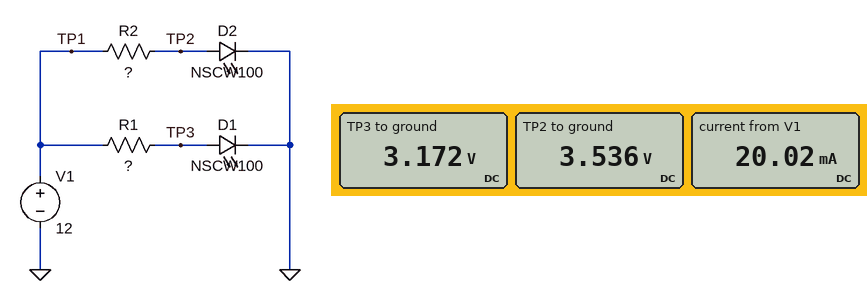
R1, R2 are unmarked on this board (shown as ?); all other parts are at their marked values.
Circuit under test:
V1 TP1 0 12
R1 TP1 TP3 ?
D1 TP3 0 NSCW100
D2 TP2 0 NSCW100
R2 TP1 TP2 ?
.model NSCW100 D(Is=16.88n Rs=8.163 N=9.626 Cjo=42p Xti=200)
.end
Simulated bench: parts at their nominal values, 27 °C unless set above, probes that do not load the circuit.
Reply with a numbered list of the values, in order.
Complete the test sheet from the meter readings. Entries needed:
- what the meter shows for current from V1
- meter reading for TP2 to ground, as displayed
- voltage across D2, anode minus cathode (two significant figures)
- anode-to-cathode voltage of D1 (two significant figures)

1. 20.02 mA
2. 3.536 V
3. 3.5 V
4. 3.2 V
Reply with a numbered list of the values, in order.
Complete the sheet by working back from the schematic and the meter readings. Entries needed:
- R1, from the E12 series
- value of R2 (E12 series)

1. 1.8 kΩ
2. 560 Ω
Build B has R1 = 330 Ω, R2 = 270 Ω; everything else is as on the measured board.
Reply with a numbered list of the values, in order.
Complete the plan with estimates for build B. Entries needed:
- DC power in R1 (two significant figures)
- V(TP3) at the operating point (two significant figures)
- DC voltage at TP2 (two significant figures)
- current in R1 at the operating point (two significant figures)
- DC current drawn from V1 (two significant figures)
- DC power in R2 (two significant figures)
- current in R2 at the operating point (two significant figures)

1. 210 mW
2. 3.7 V
3. 3.8 V
4. 25 mA
5. 55 mA
6. 250 mW
7. 30 mA
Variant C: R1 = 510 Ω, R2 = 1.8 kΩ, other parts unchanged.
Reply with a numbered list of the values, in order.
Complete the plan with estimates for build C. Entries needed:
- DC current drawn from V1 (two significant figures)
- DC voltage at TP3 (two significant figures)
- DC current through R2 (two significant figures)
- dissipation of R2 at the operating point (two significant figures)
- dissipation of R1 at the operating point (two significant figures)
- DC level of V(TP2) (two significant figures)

1. 21 mA
2. 3.6 V
3. 4.9 mA
4. 43 mW
5. 140 mW
6. 3.2 V
